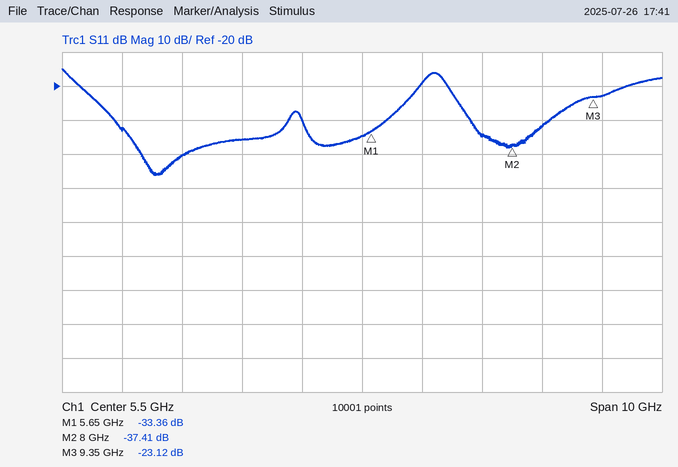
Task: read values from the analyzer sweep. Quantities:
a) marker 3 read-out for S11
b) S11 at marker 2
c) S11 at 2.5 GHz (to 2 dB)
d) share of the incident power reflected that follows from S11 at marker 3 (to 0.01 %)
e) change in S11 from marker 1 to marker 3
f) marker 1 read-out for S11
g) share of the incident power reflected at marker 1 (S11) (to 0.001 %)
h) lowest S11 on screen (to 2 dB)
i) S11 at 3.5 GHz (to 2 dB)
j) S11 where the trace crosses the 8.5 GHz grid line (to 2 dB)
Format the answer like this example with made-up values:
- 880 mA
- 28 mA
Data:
- -23.12 dB
- -37.41 dB
- -40 dB
- 0.49 %
- 10.24 dB
- -33.36 dB
- 0.046 %
- -46 dB
- -36 dB
- -32 dB
